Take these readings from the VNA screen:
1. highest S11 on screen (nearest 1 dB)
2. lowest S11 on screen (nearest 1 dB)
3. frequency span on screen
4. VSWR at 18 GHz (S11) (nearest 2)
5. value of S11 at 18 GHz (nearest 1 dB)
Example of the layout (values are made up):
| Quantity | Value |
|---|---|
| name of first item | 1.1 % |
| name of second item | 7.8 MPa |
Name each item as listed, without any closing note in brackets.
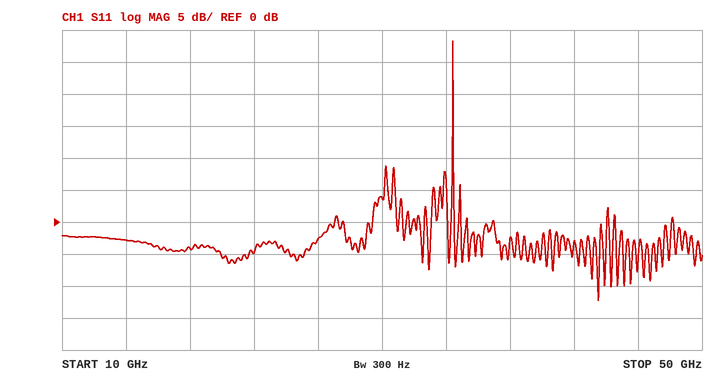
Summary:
| Quantity | Value |
|---|---|
| highest S11 on screen | 28 dB |
| lowest S11 on screen | -12 dB |
| frequency span on screen | 40 GHz |
| VSWR at 18 GHz (S11) | 4 |
| value of S11 at 18 GHz | -4 dB |
